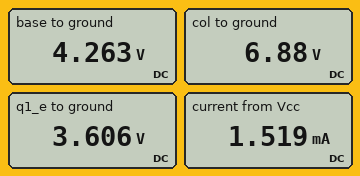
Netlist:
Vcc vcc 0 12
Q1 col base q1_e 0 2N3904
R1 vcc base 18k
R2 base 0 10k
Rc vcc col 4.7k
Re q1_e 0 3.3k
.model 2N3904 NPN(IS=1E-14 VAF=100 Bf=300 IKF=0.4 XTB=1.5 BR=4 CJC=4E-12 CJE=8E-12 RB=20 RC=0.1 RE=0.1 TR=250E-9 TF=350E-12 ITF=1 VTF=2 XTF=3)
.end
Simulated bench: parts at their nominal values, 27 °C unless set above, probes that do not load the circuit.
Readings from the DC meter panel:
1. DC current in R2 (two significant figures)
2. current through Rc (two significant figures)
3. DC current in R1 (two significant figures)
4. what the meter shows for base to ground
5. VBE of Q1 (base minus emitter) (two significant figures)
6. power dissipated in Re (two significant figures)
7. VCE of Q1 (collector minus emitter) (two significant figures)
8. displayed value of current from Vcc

430 µA
1.1 mA
430 µA
4.263 V
660 mV
3.9 mW
3.3 V
1.519 mA
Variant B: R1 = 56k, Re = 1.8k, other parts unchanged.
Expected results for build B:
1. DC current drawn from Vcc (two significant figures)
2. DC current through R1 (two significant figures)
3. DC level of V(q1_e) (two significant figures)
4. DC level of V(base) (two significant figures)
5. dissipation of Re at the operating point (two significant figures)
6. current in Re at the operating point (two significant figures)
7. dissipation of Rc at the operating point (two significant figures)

820 µA
180 µA
1.2 V
1.8 V
750 µW
640 µA
1.9 mW
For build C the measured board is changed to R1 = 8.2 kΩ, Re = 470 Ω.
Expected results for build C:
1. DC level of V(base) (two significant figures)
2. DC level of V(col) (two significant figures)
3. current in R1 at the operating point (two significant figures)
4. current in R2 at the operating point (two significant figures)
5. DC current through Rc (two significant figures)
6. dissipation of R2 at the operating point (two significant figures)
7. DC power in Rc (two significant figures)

2.2 V
1.5 V
1.2 mA
220 µA
2.2 mA
500 µW
23 mW
